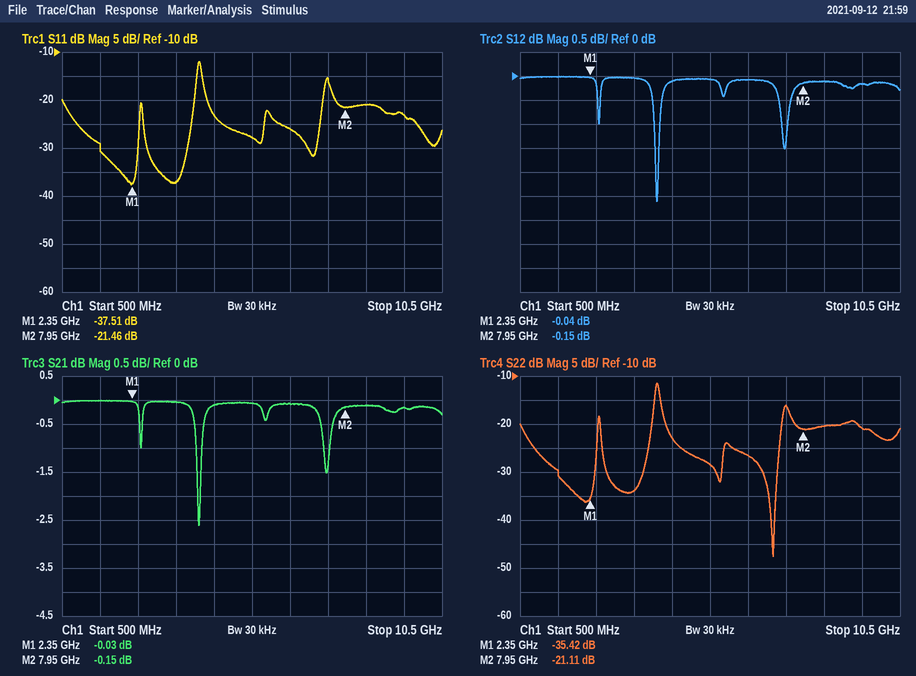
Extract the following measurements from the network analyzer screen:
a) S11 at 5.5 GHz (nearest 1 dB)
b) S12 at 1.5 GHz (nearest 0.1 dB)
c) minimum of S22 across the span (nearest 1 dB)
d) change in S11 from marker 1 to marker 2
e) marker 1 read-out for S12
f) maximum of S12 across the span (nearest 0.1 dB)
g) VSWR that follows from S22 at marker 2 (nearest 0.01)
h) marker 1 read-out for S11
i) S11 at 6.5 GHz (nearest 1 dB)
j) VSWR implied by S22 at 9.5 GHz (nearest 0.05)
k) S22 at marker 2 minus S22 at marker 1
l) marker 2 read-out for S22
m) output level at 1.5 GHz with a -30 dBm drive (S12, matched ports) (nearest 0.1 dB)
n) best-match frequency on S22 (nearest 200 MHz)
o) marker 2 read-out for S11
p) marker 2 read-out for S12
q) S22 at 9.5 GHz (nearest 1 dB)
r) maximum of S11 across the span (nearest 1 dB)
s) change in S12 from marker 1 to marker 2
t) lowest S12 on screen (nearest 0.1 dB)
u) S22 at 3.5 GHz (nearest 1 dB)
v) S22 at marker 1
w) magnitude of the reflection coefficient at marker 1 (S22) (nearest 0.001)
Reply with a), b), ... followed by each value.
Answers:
a) -28 dB
b) 0.0 dB
c) -48 dB
d) 16.05 dB
e) -0.04 dB
f) 0.0 dB
g) 1.19
h) -37.51 dB
i) -26 dB
j) 1.20
k) 14.31 dB
l) -21.11 dB
m) -30.0 dBm
n) 7.2 GHz
o) -21.46 dB
p) -0.15 dB
q) -21 dB
r) -12 dB
s) -0.11 dB
t) -2.6 dB
u) -34 dB
v) -35.42 dB
w) 0.017
